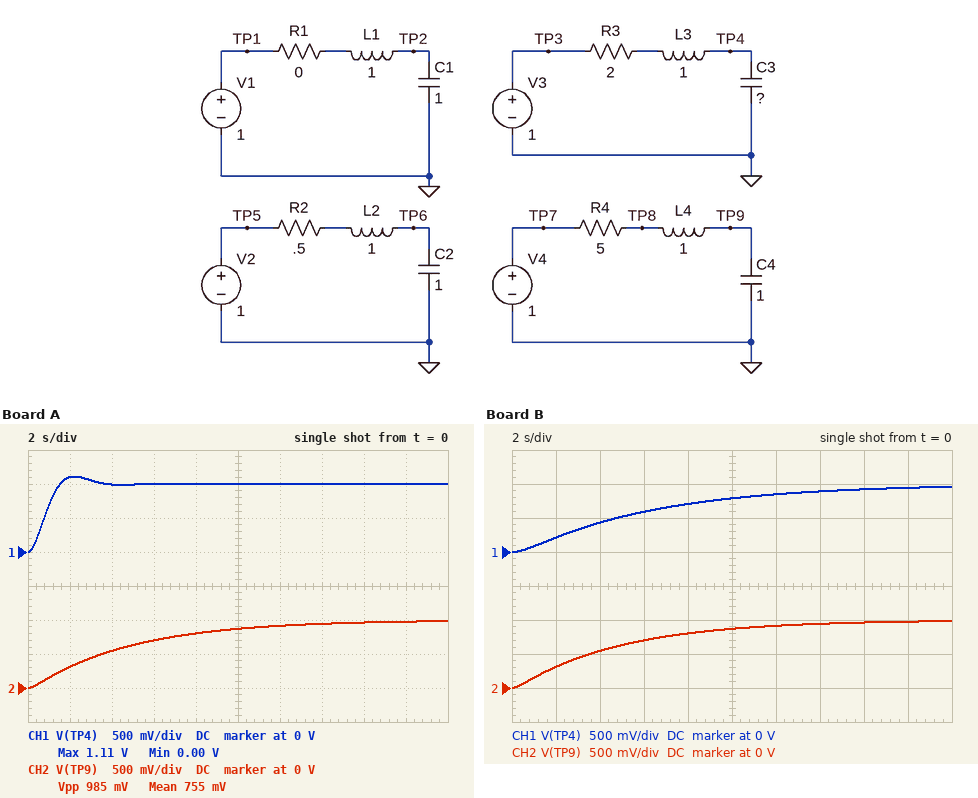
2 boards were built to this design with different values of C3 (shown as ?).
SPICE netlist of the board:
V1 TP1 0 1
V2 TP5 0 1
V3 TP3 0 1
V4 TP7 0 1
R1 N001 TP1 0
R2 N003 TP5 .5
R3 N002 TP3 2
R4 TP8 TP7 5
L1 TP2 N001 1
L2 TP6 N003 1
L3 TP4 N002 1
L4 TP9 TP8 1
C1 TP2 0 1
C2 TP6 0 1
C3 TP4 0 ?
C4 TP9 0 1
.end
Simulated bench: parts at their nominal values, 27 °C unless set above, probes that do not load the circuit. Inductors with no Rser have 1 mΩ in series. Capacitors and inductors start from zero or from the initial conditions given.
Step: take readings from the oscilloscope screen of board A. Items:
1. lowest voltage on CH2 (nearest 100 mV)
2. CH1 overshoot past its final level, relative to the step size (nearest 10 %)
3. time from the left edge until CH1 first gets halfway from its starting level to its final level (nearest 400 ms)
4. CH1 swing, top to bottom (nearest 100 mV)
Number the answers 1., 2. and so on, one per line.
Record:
1. 0 V
2. 10 %
3. 800 ms
4. 1.1 V
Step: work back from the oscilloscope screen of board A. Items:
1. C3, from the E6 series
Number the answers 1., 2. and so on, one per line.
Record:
1. 330 mF
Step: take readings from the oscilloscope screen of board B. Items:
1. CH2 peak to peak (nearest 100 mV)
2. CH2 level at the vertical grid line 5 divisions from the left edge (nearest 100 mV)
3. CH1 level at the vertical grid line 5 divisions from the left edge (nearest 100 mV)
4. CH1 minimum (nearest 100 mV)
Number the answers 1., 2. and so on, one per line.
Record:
1. 1.0 V
2. 900 mV
3. 800 mV
4. 0 V
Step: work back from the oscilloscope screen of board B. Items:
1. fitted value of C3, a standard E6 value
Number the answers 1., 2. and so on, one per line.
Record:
1. 3.3 F
